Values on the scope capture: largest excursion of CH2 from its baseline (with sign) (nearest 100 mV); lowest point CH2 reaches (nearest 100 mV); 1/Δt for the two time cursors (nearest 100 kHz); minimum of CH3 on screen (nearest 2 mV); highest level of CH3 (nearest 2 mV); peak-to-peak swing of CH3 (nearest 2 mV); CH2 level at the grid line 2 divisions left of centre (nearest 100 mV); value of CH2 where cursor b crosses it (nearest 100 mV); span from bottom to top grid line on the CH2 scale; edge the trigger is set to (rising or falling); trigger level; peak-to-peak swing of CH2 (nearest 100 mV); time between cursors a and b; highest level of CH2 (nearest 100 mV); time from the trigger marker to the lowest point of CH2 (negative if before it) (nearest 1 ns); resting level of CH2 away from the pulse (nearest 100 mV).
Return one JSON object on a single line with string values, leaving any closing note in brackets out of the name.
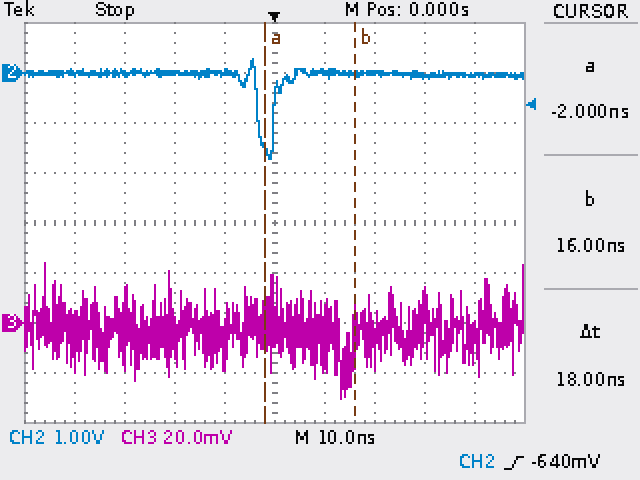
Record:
{"largest excursion of CH2 from its baseline (with sign)": "-1.7 V", "lowest point CH2 reaches": "-1.7 V", "1/Δt for the two time cursors": "55.6 MHz", "minimum of CH3 on screen": "-30 mV", "highest level of CH3": "24 mV", "peak-to-peak swing of CH3": "54 mV", "CH2 level at the grid line 2 divisions left of centre": "0.0 V", "value of CH2 where cursor b crosses it": "0.0 V", "span from bottom to top grid line on the CH2 scale": "8 V", "edge the trigger is set to": "rising", "trigger level": "-640 mV", "peak-to-peak swing of CH2": "2.0 V", "time between cursors a and b": "18 ns", "highest level of CH2": "300 mV", "time from the trigger marker to the lowest point of CH2 (negative if before it)": "-1 ns", "resting level of CH2 away from the pulse": "0.0 V"}
